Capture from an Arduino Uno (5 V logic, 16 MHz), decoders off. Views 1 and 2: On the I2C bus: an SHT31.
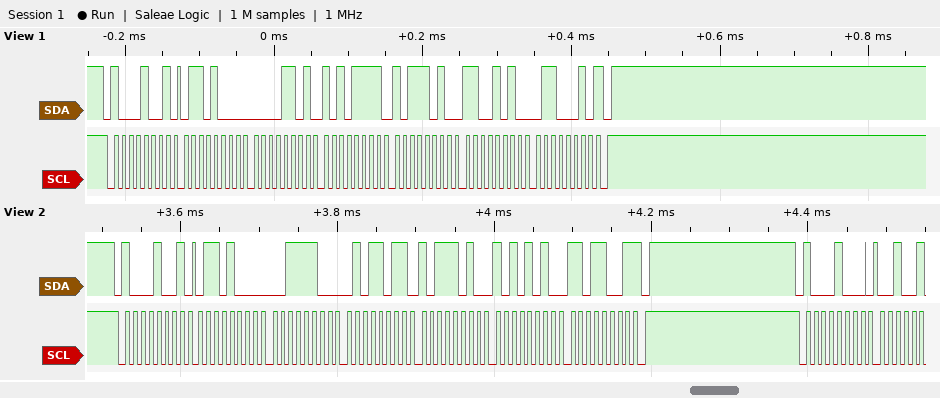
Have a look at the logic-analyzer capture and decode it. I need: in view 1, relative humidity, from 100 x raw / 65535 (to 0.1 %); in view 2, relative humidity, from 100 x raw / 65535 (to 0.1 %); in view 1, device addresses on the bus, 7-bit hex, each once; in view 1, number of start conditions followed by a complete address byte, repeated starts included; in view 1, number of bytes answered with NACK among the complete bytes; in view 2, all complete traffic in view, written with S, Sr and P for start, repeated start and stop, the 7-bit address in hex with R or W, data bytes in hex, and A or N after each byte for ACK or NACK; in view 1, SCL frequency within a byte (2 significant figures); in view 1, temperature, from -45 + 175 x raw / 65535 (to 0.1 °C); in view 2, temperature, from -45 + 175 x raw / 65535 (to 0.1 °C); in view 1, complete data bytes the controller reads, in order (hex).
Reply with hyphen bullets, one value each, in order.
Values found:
- 73.0 %
- 72.9 %
- 0x44
- 1
- 1
- S 44R A 68 A 3C A 5B A BA A AA A D9 N P S 44W A
- 100 kHz
- 26.1 °C
- 26.3 °C
- 68 0D AF BA CA 62
